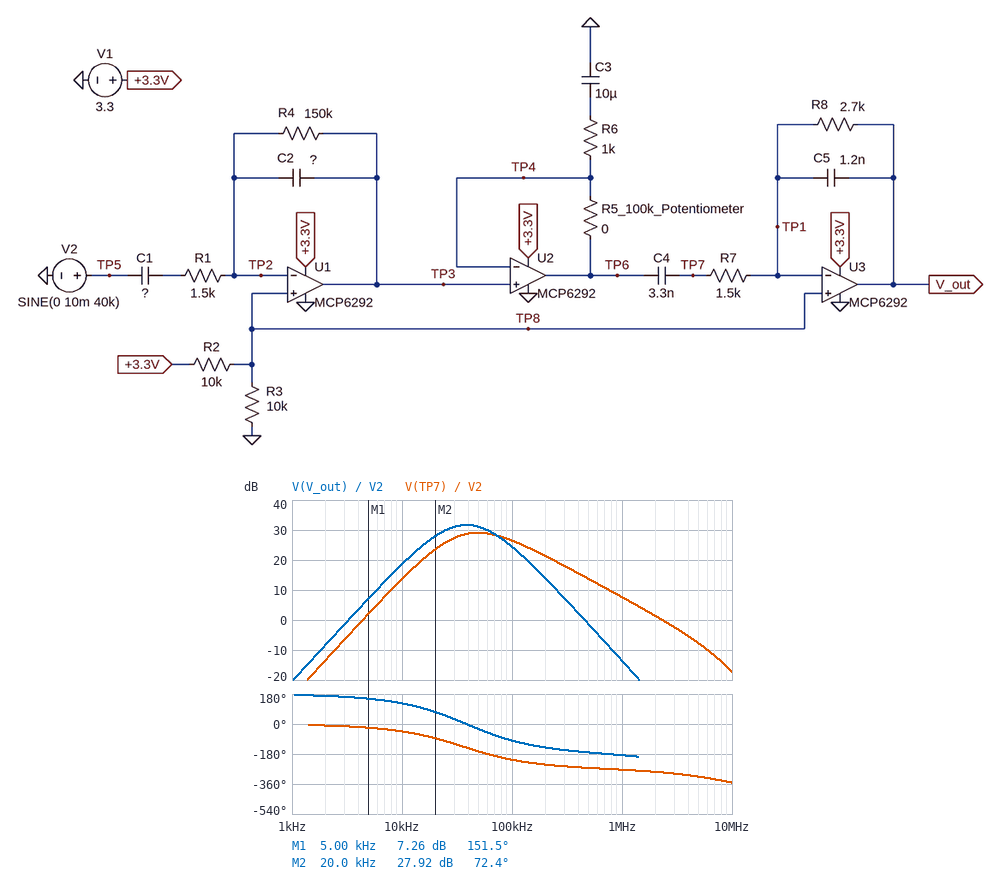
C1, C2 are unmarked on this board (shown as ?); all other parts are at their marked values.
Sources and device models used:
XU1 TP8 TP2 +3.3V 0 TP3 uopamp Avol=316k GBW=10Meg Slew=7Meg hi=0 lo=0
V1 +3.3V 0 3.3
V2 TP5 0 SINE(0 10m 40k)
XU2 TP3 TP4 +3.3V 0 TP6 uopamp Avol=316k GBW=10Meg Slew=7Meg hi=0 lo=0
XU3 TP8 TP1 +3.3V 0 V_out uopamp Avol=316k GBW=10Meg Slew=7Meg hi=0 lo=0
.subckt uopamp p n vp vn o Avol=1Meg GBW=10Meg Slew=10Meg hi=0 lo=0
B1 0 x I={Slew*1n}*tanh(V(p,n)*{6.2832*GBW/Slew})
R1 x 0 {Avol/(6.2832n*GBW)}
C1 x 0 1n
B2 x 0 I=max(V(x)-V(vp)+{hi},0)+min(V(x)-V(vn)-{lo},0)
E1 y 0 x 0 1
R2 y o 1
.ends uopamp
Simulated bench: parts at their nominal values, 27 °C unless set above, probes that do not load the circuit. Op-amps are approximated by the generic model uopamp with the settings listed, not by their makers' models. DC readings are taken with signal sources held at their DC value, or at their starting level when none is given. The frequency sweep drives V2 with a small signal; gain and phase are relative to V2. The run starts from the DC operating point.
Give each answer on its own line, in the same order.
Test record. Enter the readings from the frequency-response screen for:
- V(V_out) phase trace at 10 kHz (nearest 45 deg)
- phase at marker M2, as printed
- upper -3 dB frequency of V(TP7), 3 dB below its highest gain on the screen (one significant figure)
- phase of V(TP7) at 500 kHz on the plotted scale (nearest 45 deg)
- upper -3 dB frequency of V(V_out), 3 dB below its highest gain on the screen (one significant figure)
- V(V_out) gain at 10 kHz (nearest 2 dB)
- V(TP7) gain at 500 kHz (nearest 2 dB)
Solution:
135 deg
72.4 deg
100 kHz
-270 deg
70 kHz
18 dB
14 dB
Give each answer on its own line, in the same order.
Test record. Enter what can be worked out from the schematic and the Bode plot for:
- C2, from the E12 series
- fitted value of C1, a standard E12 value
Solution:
33 pF
1.8 nF
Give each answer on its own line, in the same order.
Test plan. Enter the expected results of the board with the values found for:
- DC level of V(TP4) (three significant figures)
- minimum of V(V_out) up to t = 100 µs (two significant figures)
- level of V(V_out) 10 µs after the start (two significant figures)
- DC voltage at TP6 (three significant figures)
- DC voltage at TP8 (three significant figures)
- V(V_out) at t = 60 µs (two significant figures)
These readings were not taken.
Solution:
1.65 V
1.3 V
1.8 V
1.65 V
1.65 V
1.9 V
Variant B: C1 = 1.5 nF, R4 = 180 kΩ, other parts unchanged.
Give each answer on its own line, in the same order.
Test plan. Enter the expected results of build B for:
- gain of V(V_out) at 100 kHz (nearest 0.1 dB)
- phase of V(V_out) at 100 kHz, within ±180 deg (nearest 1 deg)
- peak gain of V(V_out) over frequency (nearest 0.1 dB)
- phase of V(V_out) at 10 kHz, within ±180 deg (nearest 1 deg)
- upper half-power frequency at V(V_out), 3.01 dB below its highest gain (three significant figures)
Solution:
24.2 dB
-97 deg
31.1 dB
122 deg
70.7 kHz
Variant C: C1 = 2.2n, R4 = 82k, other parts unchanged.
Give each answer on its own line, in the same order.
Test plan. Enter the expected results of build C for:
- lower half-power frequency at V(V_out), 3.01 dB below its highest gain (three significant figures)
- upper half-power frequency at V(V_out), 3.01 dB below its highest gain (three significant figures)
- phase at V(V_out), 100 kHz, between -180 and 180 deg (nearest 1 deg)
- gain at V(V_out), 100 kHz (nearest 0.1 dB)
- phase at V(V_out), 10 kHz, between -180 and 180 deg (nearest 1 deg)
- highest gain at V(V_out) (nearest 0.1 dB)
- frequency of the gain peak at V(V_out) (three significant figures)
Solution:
24.3 kHz
76.7 kHz
-92 deg
24.2 dB
129 deg
30.2 dB
43.3 kHz
